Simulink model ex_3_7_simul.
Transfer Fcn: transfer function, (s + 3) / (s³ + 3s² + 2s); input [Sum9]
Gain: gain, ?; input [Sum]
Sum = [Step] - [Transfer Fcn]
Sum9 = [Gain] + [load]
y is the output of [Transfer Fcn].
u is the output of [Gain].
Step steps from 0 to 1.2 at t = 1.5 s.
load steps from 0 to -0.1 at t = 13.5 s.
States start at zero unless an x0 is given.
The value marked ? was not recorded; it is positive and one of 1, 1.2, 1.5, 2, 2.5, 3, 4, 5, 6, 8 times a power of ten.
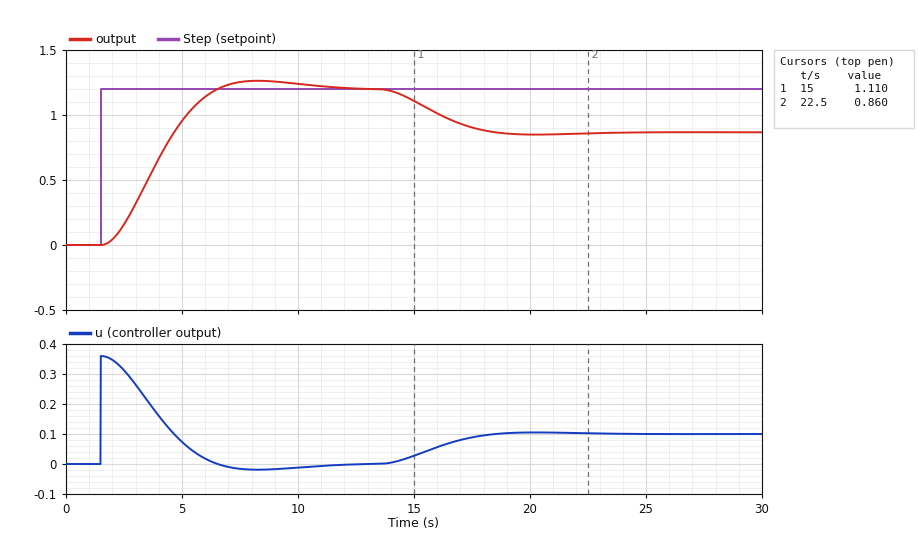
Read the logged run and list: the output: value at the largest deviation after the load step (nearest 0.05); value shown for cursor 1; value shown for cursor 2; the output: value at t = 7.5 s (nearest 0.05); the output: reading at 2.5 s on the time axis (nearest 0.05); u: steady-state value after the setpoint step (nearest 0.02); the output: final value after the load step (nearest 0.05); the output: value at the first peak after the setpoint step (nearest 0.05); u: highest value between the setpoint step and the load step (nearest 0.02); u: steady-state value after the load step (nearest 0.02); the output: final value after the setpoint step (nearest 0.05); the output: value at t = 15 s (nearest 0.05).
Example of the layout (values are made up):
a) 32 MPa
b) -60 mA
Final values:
a) 0.85
b) 1.110
c) 0.860
d) 1.25
e) 0.15
f) 0.00
g) 0.85
h) 1.25
i) 0.36
j) 0.10
k) 1.20
l) 1.10
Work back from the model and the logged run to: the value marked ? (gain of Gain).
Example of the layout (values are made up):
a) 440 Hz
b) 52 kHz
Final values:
a) 0.3
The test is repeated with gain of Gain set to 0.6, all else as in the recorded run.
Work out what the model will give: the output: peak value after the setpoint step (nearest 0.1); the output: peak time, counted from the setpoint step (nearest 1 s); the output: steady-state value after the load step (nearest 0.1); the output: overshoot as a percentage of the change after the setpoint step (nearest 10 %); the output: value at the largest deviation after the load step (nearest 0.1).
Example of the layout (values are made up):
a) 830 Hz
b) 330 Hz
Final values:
a) 1.4
b) 4 s
c) 1.0
d) 20 %
e) 1.0
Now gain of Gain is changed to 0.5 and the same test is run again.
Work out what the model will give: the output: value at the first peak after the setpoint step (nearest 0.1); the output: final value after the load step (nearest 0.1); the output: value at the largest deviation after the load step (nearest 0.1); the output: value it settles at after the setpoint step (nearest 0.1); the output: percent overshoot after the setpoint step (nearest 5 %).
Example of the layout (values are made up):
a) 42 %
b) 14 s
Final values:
a) 1.4
b) 1.0
c) 1.0
d) 1.2
e) 15 %
